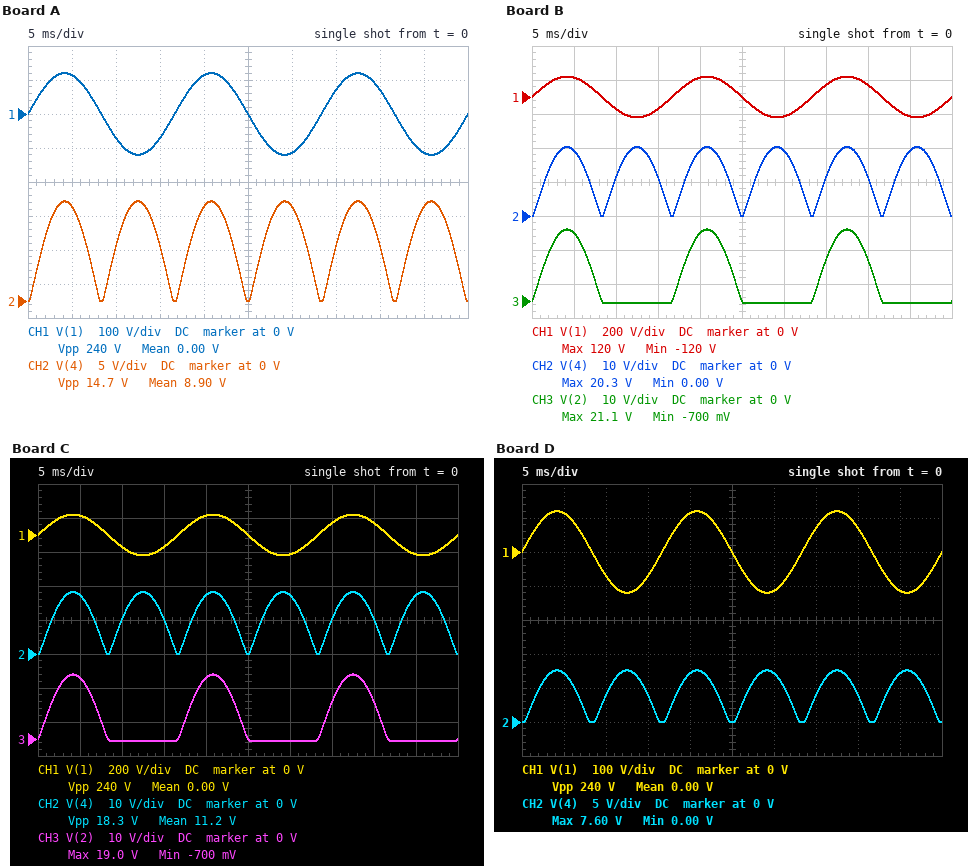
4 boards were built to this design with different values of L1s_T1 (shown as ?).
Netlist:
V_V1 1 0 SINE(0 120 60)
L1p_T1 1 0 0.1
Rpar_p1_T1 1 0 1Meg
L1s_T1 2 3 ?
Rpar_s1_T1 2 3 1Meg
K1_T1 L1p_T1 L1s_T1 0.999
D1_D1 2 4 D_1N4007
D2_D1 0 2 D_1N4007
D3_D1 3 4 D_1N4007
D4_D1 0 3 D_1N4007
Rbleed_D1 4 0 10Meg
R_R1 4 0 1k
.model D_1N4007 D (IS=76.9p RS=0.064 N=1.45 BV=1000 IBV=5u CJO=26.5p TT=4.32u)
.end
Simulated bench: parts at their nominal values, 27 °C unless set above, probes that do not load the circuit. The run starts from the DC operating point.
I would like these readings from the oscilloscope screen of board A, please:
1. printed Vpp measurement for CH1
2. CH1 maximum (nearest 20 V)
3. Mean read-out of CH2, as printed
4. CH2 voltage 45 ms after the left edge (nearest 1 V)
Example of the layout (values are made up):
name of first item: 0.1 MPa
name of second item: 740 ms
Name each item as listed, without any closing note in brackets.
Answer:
printed Vpp measurement for CH1: 240 V
CH1 maximum: 120 V
Mean read-out of CH2, as printed: 8.90 V
CH2 voltage 45 ms after the left edge: 14 V
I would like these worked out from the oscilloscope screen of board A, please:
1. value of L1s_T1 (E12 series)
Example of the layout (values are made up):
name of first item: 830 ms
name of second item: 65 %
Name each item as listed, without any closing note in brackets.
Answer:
value of L1s_T1: 1.8 mH
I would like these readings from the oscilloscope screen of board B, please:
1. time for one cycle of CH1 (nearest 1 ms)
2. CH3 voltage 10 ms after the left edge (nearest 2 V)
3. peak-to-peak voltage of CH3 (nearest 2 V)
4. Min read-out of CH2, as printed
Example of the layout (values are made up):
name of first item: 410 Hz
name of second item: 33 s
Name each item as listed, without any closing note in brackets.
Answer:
time for one cycle of CH1: 17 ms
CH3 voltage 10 ms after the left edge: 0 V
peak-to-peak voltage of CH3: 22 V
Min read-out of CH2, as printed: 0.00 V
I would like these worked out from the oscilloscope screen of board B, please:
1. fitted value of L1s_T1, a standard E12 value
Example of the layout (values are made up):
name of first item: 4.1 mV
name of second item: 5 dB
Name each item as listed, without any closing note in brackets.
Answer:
fitted value of L1s_T1, a standard E12 value: 3.3 mH
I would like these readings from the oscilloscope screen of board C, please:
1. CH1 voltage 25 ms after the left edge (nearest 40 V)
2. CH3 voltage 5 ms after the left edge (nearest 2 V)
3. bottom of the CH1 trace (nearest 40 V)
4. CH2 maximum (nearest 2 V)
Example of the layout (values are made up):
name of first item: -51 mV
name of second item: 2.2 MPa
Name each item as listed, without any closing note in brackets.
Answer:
CH1 voltage 25 ms after the left edge: 0 V
CH3 voltage 5 ms after the left edge: 18 V
bottom of the CH1 trace: -120 V
CH2 maximum: 18 V
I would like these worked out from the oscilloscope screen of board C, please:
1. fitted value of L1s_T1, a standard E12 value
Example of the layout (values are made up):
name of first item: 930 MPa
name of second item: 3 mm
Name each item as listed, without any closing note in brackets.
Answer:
fitted value of L1s_T1, a standard E12 value: 2.7 mH
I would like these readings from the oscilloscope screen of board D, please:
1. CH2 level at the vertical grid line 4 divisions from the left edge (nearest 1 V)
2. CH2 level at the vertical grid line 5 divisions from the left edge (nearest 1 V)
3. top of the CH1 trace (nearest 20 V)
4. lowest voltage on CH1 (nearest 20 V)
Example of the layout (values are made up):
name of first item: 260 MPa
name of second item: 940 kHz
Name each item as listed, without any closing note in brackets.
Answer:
CH2 level at the vertical grid line 4 divisions from the left edge: 7 V
CH2 level at the vertical grid line 5 divisions from the left edge: 0 V
top of the CH1 trace: 120 V
lowest voltage on CH1: -120 V
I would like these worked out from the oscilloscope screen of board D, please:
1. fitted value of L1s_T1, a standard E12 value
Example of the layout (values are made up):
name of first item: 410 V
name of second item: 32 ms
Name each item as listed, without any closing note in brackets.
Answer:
fitted value of L1s_T1, a standard E12 value: 560 µH
